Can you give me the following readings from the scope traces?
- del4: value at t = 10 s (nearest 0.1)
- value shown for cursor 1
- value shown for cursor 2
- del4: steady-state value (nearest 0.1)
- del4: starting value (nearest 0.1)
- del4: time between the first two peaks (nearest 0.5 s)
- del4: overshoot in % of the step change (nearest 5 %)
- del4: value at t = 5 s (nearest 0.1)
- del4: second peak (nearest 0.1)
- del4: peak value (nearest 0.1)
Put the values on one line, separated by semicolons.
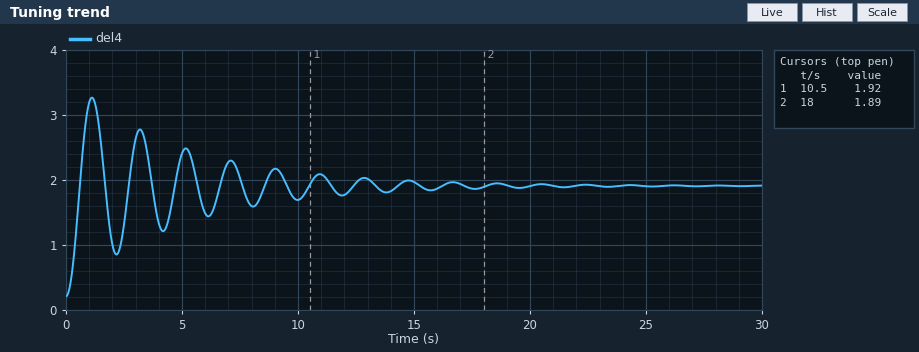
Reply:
1.7; 1.92; 1.89; 1.9; 0.2; 2.0 s; 80 %; 2.4; 2.8; 3.3
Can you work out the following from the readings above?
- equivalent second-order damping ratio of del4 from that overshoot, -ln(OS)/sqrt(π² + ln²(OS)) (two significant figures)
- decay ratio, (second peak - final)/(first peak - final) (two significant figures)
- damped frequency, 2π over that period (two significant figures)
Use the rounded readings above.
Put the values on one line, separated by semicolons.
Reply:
0.071; 0.64; 3.1 rad/s
